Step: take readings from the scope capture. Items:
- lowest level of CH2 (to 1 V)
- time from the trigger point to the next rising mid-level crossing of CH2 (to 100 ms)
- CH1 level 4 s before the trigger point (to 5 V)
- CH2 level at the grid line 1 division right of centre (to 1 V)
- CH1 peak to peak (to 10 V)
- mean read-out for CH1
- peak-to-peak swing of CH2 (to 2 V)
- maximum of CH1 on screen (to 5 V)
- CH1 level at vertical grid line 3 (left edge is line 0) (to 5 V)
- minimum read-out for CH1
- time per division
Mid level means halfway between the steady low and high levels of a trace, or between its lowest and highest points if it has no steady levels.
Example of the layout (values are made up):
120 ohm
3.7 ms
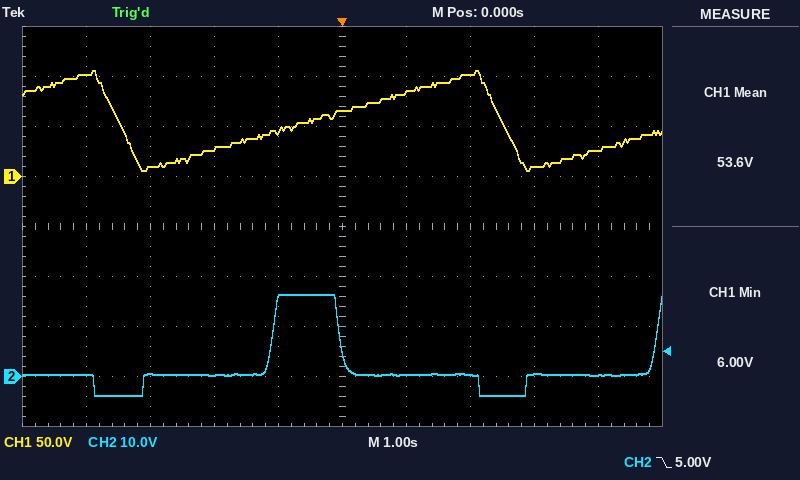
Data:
-4 V
4.9 s
100 V
0 V
100 V
53.6 V
20 V
105 V
30 V
6.00 V
1 s
